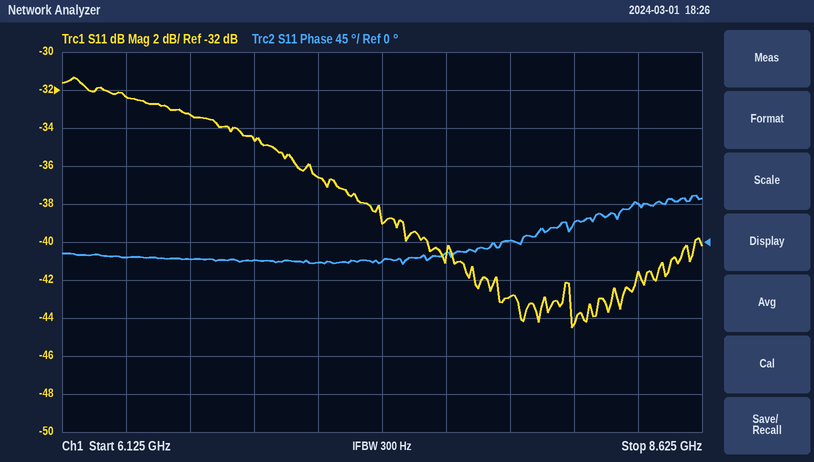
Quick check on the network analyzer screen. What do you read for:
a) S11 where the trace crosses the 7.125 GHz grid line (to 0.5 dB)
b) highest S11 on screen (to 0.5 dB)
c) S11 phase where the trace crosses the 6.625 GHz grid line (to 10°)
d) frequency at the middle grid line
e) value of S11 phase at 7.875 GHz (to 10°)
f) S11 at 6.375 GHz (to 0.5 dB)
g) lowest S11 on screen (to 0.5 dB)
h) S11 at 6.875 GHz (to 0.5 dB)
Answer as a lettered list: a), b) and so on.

a) -36.5 dB
b) -31.5 dB
c) -20°
d) 7.375 GHz
e) 0°
f) -32.5 dB
g) -44.5 dB
h) -34.5 dB
